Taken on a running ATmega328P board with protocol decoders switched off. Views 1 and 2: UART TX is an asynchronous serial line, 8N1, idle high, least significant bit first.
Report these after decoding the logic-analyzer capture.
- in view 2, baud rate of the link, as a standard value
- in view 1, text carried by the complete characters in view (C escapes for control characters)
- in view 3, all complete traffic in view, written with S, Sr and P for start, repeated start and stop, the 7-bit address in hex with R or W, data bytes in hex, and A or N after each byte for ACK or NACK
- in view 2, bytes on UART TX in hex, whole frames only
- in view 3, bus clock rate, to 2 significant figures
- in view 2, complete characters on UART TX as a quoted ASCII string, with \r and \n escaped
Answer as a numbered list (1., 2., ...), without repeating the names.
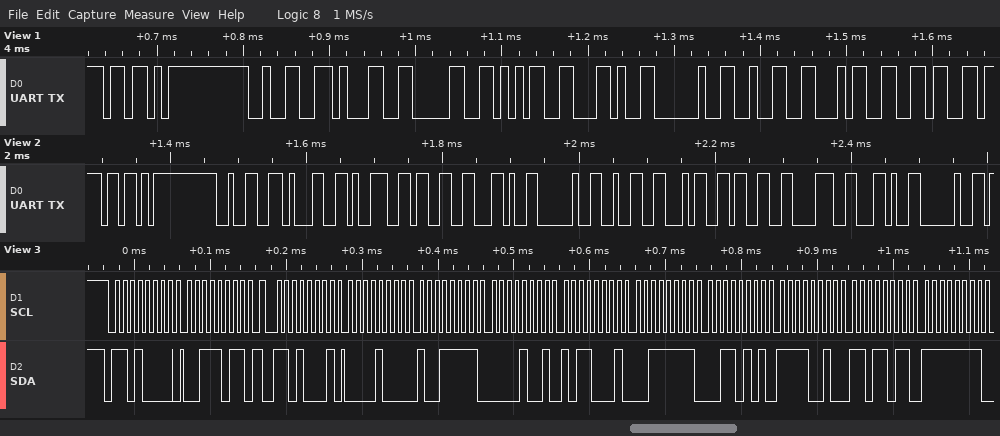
1. 115200 baud
2. "[2105, 246"
3. S 68W A 3B A Sr 68R A 08 A 9F A 09 A B1 A 3F A 35 A F2 A DB A FF A
4. 0x5B 0x32 0x31 0x39 0x33 0x2C 0x20 0x32 0x34 0x33 0x38 0x2C 0x20
5. 100 kHz
6. "[2193, 2438, "
